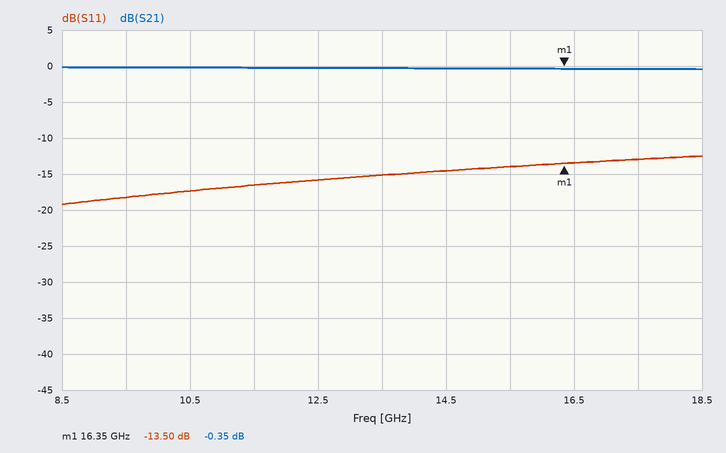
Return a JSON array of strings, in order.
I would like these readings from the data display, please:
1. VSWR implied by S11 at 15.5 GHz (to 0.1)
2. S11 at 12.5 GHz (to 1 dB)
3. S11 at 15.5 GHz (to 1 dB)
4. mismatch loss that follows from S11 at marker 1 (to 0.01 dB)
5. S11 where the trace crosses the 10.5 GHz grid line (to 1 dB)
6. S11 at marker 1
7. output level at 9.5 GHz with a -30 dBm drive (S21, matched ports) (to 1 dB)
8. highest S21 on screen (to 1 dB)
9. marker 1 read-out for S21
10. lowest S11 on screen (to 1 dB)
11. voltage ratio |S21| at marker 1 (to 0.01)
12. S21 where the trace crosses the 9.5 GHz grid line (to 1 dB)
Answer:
["1.5", "-16 dB", "-14 dB", "0.20 dB", "-17 dB", "-13.50 dB", "-30 dBm", "0 dB", "-0.35 dB", "-19 dB", "0.96", "0 dB"]
